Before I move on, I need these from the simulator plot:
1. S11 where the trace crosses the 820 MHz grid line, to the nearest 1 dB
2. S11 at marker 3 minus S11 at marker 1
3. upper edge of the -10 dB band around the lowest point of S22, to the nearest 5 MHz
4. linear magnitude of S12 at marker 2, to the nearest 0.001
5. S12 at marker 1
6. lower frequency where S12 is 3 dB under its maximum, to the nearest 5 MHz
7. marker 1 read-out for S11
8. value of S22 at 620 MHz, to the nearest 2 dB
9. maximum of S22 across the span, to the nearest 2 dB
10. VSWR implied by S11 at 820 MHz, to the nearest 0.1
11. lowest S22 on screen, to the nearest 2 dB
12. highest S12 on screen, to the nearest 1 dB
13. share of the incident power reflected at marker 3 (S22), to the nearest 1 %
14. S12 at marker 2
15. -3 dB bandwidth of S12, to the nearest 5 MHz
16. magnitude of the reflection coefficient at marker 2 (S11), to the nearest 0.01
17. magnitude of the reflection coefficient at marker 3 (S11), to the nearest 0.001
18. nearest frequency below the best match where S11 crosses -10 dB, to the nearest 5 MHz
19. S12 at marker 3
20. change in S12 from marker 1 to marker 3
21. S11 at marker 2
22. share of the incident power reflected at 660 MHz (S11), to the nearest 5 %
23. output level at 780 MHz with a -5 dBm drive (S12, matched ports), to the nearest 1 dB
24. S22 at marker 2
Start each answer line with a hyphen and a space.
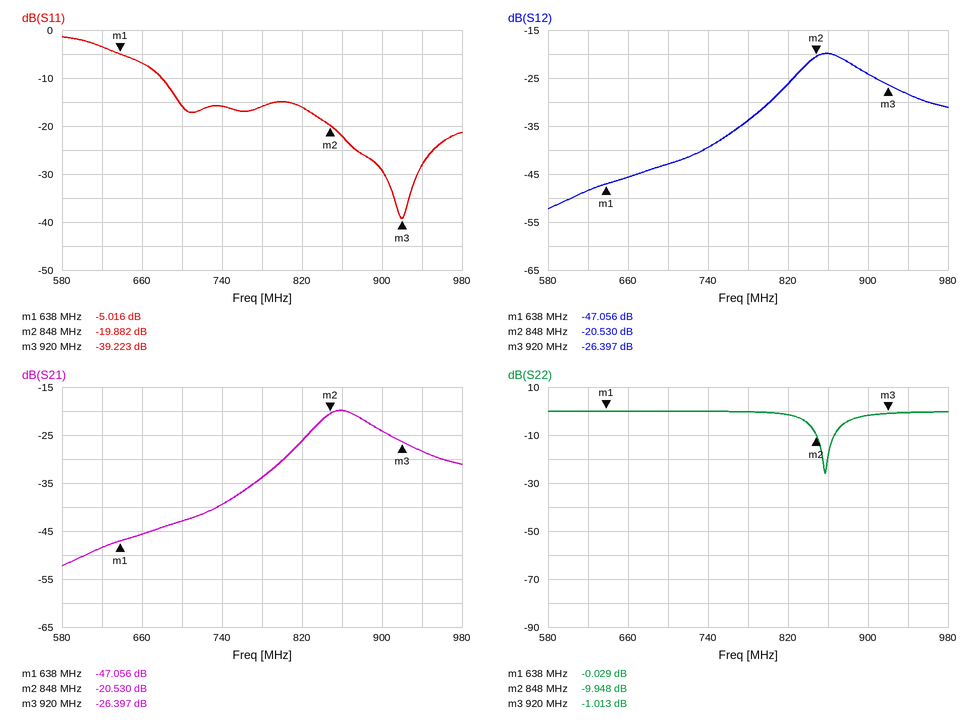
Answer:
- -16 dB
- -34.207 dB
- 865 MHz
- 0.094
- -47.056 dB
- 835 MHz
- -5.016 dB
- 0 dB
- 0 dB
- 1.4
- -26 dB
- -20 dB
- 79 %
- -20.530 dB
- 55 MHz
- 0.10
- 0.011
- 680 MHz
- -26.397 dB
- 20.659 dB
- -19.882 dB
- 20 %
- -39 dBm
- -9.948 dB
